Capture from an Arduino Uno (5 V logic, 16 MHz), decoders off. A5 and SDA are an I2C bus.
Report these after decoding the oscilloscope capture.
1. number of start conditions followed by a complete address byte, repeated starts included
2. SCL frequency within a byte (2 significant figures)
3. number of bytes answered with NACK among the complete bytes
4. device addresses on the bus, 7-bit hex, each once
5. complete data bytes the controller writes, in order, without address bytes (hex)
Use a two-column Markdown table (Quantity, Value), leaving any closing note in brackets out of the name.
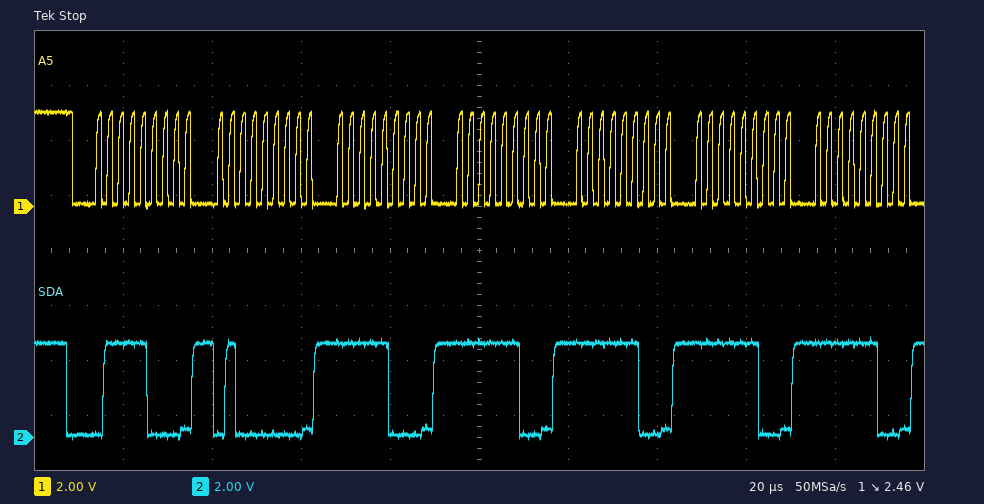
| Quantity | Value |
|---|---|
| number of start conditions followed by a complete address byte, repeated starts included | 1 |
| SCL frequency within a byte | 400 kHz |
| number of bytes answered with NACK among the complete bytes | 0 |
| device addresses on the bus, 7-bit hex, each once | 0x3C |
| complete data bytes the controller writes, in order, without address bytes | 40 F8 FC FC FC FC |
